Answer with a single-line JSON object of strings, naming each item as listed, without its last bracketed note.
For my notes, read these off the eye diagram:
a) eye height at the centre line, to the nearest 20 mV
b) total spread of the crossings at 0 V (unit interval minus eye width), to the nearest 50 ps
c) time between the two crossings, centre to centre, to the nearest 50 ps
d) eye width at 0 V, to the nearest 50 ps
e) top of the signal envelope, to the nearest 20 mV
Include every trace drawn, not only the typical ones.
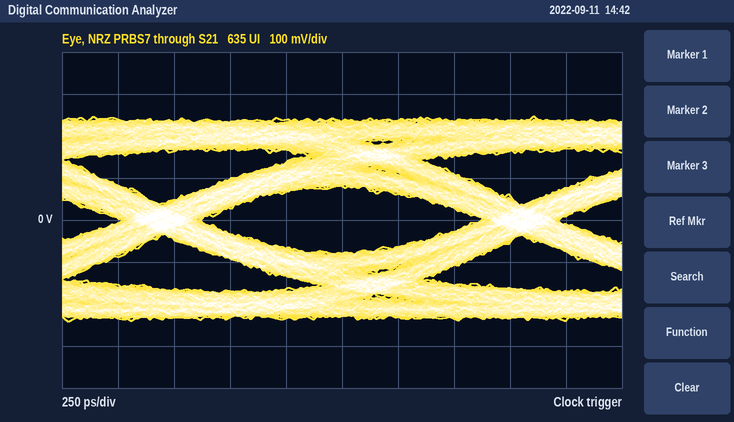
{"eye height at the centre line, to the nearest 20 mV": "160 mV", "total spread of the crossings at 0 V (unit interval minus eye width), to the nearest 50 ps": "350 ps", "time between the two crossings, centre to centre, to the nearest 50 ps": "1.60 ns", "eye width at 0 V, to the nearest 50 ps": "1.25 ns", "top of the signal envelope, to the nearest 20 mV": "240 mV"}
